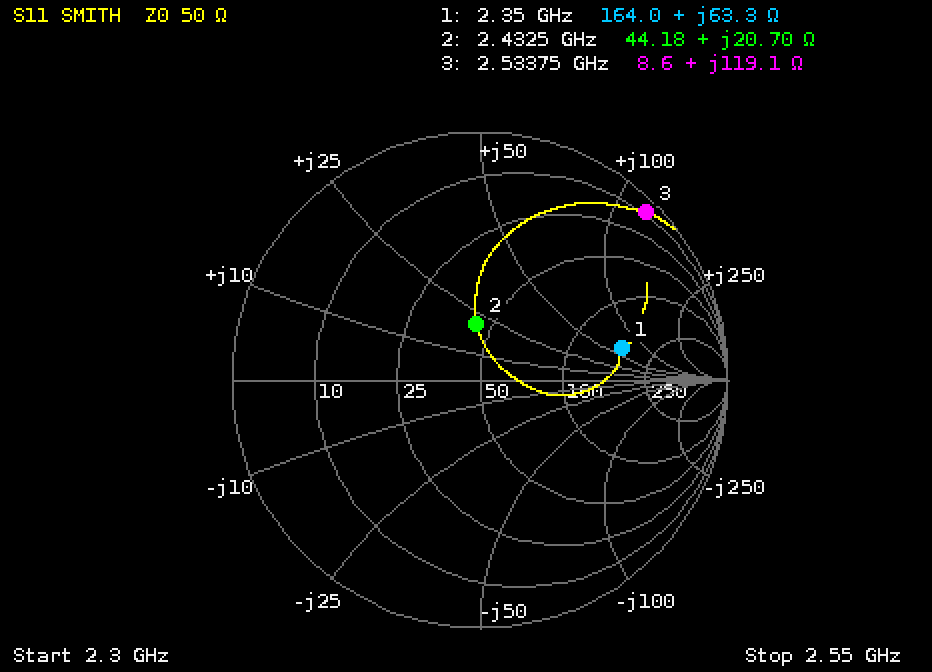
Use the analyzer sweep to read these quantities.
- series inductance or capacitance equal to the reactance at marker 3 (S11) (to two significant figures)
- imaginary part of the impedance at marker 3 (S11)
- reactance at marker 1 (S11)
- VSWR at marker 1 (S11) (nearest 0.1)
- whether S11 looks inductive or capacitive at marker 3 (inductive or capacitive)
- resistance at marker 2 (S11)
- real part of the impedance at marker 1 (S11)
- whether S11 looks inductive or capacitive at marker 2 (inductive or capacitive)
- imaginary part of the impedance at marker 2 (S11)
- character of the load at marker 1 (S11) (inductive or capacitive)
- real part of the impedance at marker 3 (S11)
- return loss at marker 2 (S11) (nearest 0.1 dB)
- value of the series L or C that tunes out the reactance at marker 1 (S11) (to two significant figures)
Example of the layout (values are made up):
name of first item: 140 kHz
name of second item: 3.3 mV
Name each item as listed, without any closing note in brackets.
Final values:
series inductance or capacitance equal to the reactance at marker 3 (S11): 7.5 nH
imaginary part of the impedance at marker 3: +119.1 Ω
reactance at marker 1: +63.3 Ω
VSWR at marker 1 (S11): 3.8
whether S11 looks inductive or capacitive at marker 3: inductive
resistance at marker 2: 44.18 Ω
real part of the impedance at marker 1: 164.0 Ω
whether S11 looks inductive or capacitive at marker 2: inductive
imaginary part of the impedance at marker 2: +20.70 Ω
character of the load at marker 1 (S11): inductive
real part of the impedance at marker 3: 8.6 Ω
return loss at marker 2 (S11): 13.0 dB
value of the series L or C that tunes out the reactance at marker 1 (S11): 1.1 pF
